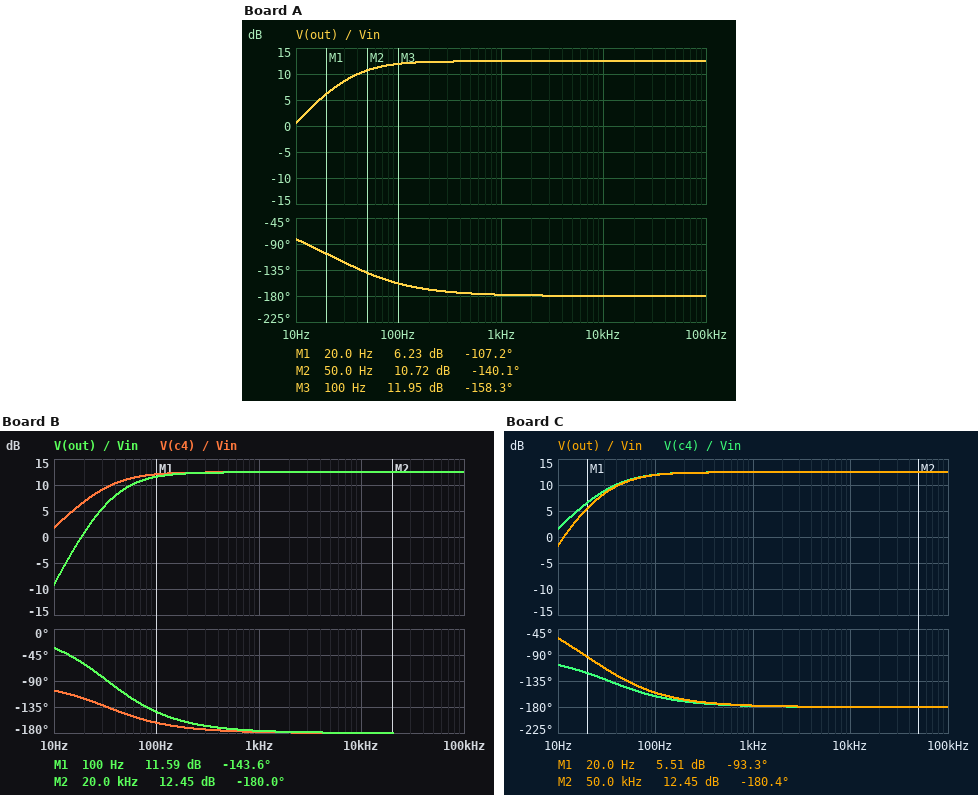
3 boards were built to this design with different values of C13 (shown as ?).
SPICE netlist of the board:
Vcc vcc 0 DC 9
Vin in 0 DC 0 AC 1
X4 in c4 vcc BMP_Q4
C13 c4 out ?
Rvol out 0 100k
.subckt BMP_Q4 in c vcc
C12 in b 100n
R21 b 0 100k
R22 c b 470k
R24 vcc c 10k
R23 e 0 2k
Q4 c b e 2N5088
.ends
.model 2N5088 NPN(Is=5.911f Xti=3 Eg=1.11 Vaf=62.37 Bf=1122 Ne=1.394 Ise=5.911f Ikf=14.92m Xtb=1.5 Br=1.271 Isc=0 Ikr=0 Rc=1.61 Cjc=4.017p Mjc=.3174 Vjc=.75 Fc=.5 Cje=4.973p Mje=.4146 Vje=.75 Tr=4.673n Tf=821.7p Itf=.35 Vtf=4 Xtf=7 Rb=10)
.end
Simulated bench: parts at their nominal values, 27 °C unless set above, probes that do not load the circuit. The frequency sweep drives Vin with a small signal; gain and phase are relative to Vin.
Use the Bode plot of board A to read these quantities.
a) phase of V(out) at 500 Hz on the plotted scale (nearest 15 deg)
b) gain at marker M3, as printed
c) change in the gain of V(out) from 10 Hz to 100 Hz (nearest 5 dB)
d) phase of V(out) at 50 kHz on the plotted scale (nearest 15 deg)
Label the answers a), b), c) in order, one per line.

a) -180 deg
b) 11.95 dB
c) 10 dB
d) -180 deg
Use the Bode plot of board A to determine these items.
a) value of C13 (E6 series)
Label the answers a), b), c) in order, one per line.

a) 330 nF
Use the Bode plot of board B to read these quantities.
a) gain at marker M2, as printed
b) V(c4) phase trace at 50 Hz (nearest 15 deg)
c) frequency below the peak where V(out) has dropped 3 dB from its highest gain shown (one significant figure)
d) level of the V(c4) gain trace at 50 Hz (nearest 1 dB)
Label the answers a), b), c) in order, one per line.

a) 12.45 dB
b) -150 deg
c) 50 Hz
d) 11 dB
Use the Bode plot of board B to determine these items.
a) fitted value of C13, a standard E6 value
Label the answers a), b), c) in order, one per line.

a) 47 nF
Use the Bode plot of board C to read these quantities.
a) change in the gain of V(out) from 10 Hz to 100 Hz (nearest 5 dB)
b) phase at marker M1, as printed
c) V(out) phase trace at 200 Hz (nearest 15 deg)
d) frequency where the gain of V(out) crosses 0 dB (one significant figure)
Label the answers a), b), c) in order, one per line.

a) 15 dB
b) -93.3 deg
c) -165 deg
d) 10 Hz
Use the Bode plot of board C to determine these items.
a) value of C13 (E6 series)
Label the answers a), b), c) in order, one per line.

a) 150 nF
